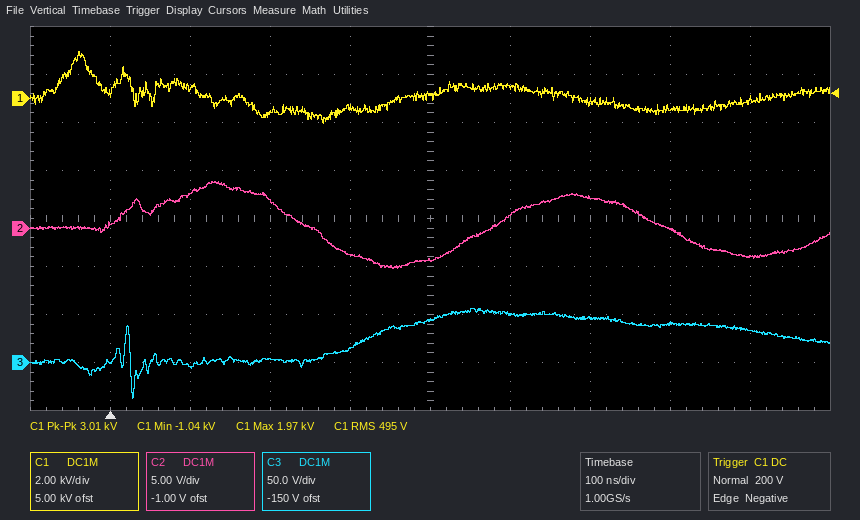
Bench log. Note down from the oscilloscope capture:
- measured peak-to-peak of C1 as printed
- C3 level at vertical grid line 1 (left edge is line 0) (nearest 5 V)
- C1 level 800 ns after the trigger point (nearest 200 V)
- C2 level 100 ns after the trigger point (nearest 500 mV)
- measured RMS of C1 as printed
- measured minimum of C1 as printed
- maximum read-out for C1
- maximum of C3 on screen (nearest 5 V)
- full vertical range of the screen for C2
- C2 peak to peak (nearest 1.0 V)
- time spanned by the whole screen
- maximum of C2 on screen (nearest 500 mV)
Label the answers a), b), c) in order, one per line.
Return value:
a) 3.01 kV
b) 0 V
c) 0.0 kV
d) 3.5 V
e) 495 V
f) -1.04 kV
g) 1.97 kV
h) 55 V
i) 40 V
j) 9.0 V
k) 1 µs
l) 5.0 V
